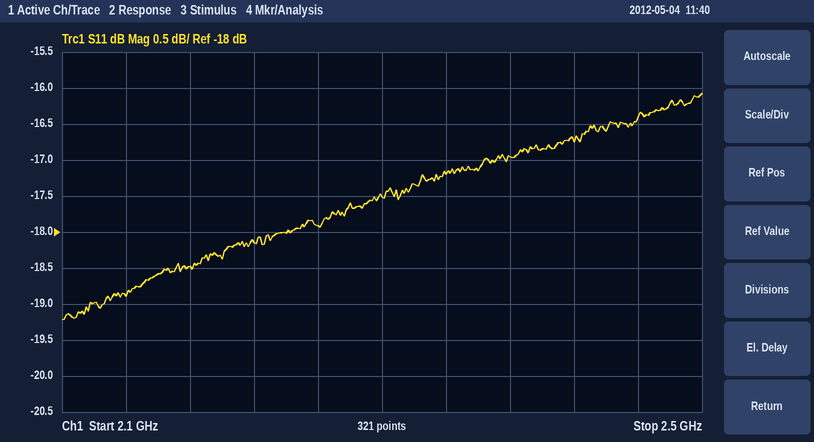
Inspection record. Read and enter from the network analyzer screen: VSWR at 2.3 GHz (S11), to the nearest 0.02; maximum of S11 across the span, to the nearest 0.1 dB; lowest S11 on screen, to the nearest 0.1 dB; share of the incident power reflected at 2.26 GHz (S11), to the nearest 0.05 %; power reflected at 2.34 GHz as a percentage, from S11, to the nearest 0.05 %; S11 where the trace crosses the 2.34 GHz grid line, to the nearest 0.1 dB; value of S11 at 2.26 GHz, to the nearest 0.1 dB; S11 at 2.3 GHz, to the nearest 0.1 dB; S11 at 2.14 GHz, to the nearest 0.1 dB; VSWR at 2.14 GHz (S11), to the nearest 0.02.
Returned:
1.30
-16.1 dB
-19.2 dB
1.60 %
1.90 %
-17.2 dB
-17.9 dB
-17.5 dB
-18.9 dB
1.26
